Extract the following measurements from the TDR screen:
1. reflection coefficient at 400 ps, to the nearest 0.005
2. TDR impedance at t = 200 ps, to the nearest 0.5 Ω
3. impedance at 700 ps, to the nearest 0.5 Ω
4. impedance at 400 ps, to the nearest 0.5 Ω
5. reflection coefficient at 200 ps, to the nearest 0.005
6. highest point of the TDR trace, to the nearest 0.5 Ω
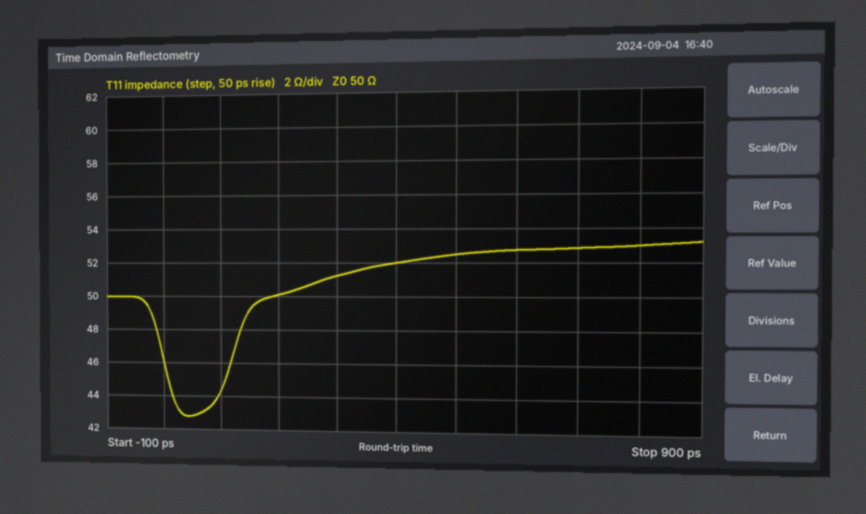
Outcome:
+0.020
50.0 Ω
53.0 Ω
52.0 Ω
0.000
53.0 Ω
